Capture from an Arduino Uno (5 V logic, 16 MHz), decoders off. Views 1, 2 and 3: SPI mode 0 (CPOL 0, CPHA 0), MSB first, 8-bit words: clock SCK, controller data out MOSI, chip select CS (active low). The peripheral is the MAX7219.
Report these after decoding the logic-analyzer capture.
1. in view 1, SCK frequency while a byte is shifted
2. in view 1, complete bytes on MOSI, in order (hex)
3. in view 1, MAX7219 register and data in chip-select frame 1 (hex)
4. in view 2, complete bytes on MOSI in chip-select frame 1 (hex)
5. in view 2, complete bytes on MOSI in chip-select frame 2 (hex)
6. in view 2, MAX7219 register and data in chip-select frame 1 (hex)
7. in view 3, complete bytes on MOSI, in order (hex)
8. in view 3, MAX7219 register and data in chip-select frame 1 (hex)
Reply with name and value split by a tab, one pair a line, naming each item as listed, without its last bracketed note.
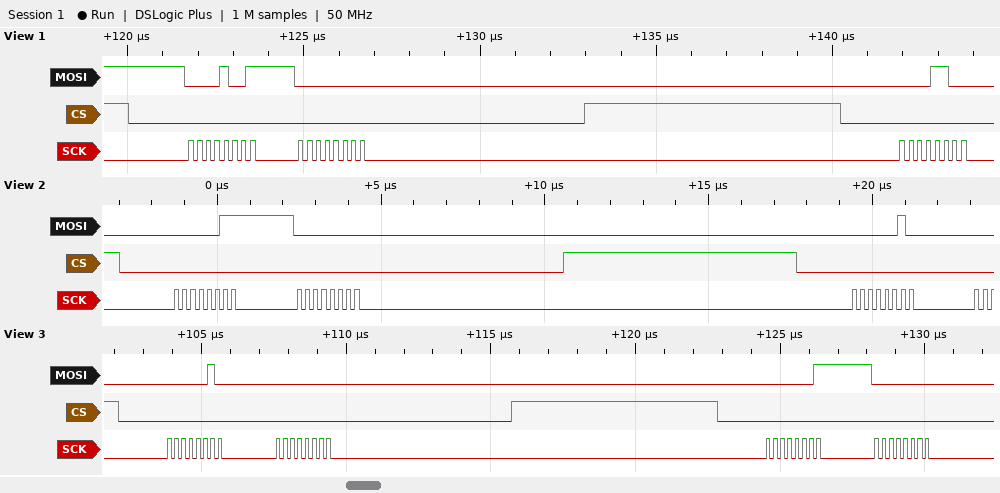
in view 1, SCK frequency while a byte is shifted	4 MHz
in view 1, complete bytes on MOSI, in order	09 00 0C
in view 1, MAX7219 register and data in chip-select frame 1	register 0x9, data 0x00
in view 2, complete bytes on MOSI in chip-select frame 1	03 00
in view 2, complete bytes on MOSI in chip-select frame 2	02
in view 2, MAX7219 register and data in chip-select frame 1	register 0x3, data 0x00
in view 3, complete bytes on MOSI, in order	02 00 01 00
in view 3, MAX7219 register and data in chip-select frame 1	register 0x2, data 0x00
